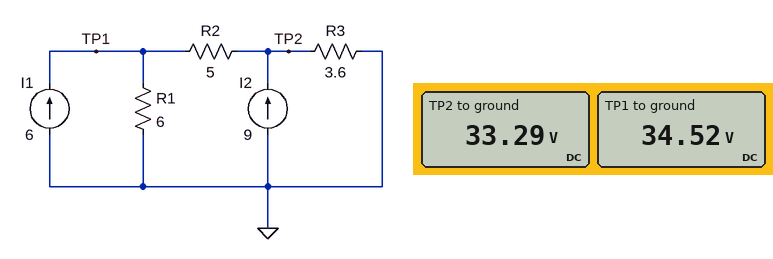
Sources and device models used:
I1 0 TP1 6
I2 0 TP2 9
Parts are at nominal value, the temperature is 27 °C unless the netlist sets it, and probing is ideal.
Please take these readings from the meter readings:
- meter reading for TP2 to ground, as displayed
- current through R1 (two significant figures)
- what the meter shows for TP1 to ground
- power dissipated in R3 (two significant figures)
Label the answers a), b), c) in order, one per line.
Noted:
a) 33.29 V
b) 5.8 A
c) 34.52 V
d) 310 W
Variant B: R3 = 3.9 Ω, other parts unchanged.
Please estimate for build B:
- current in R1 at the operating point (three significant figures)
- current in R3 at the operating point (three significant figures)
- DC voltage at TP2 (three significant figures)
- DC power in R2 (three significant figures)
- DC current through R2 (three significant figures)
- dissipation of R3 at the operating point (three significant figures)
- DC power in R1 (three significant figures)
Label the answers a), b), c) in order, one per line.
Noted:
a) 5.94 A
b) 9.06 A
c) 35.3 V
d) 18.2 mW
e) 60.4 mA
f) 320 W
g) 212 W
